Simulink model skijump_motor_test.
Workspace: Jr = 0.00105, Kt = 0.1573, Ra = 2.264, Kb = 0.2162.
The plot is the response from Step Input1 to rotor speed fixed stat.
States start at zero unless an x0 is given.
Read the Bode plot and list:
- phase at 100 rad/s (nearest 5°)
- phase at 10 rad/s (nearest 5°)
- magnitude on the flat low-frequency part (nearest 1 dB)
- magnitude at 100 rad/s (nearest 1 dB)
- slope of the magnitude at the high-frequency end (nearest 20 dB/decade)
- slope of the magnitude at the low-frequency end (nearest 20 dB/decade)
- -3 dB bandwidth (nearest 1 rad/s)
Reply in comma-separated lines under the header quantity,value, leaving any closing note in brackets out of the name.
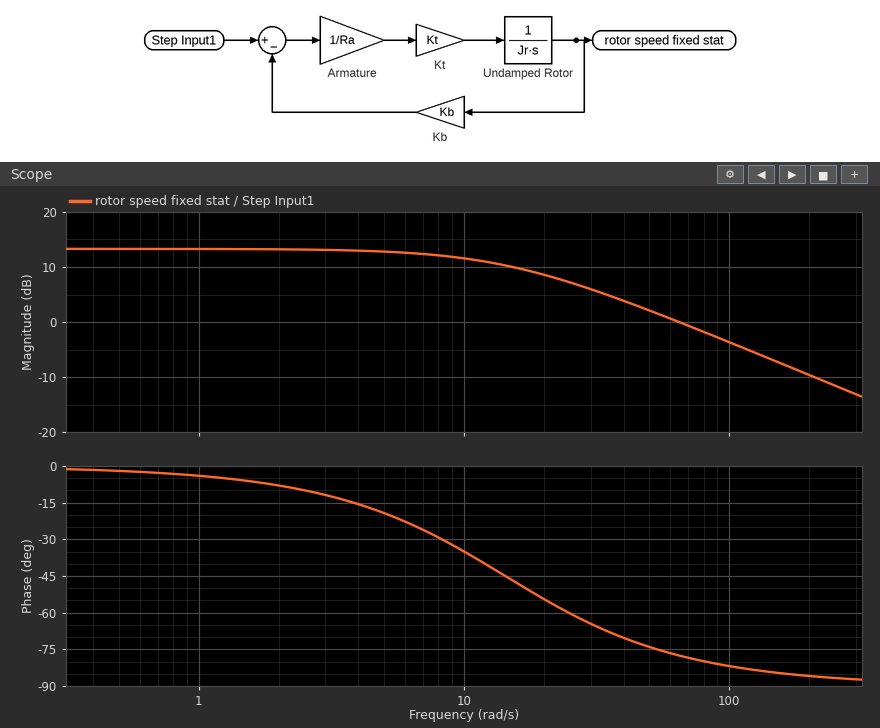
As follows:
quantity,value
phase at 100 rad/s,-80°
phase at 10 rad/s,-35°
magnitude on the flat low-frequency part,13 dB
magnitude at 100 rad/s,-4 dB
slope of the magnitude at the high-frequency end,-20 dB/decade
slope of the magnitude at the low-frequency end,0 dB/decade
-3 dB bandwidth,14 rad/s
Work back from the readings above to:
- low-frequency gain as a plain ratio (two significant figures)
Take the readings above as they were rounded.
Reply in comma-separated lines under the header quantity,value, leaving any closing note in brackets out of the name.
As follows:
quantity,value
low-frequency gain as a plain ratio,4.5
